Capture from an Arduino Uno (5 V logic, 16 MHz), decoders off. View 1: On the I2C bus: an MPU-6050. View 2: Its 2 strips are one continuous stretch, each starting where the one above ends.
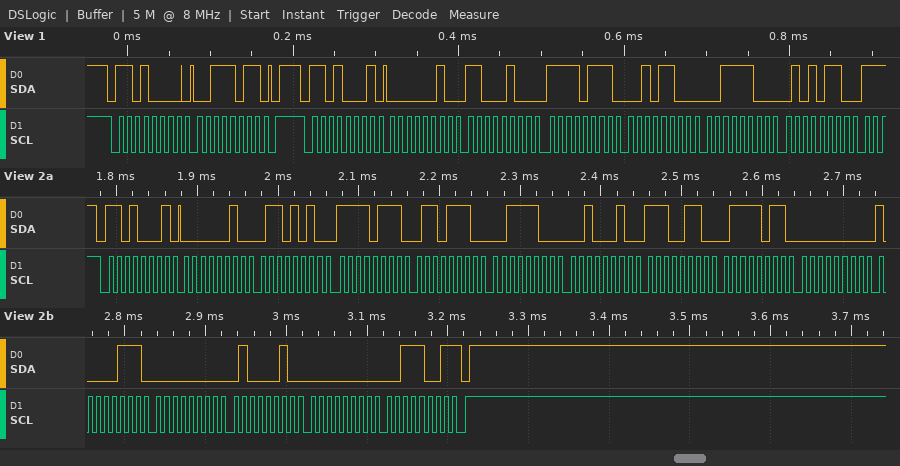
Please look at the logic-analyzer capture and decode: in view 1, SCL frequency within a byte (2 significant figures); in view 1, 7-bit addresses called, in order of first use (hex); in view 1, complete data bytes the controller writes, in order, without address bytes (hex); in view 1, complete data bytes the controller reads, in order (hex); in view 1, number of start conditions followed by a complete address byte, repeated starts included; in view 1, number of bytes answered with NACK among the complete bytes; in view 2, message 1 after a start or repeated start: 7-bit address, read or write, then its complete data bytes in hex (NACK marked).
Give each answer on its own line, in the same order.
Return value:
100 kHz
0x68
3B
02 C4 F7 2C 3C 56
2
0
0x68 read: 02 6A F7 6E 3C 22 E6 7B 00 87 00 42 00 39 NACK
